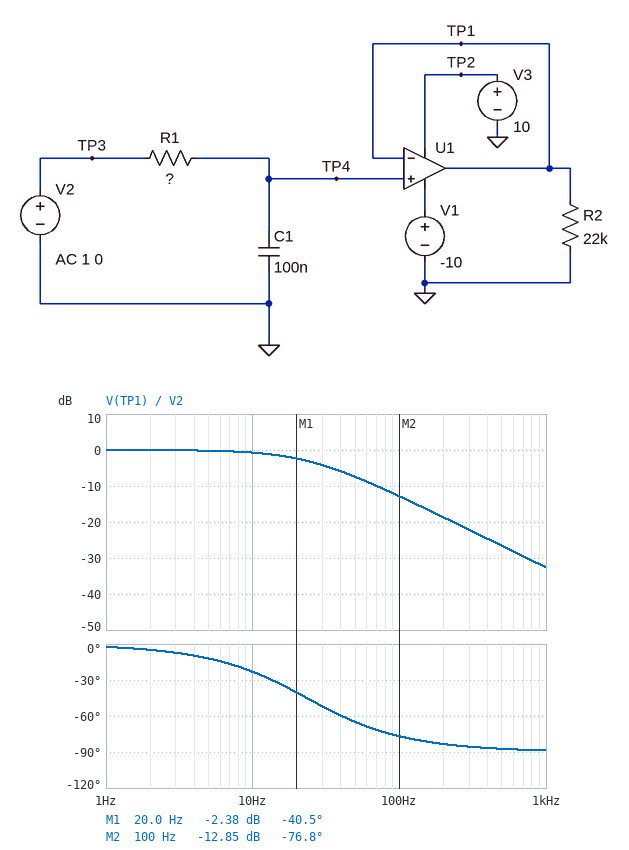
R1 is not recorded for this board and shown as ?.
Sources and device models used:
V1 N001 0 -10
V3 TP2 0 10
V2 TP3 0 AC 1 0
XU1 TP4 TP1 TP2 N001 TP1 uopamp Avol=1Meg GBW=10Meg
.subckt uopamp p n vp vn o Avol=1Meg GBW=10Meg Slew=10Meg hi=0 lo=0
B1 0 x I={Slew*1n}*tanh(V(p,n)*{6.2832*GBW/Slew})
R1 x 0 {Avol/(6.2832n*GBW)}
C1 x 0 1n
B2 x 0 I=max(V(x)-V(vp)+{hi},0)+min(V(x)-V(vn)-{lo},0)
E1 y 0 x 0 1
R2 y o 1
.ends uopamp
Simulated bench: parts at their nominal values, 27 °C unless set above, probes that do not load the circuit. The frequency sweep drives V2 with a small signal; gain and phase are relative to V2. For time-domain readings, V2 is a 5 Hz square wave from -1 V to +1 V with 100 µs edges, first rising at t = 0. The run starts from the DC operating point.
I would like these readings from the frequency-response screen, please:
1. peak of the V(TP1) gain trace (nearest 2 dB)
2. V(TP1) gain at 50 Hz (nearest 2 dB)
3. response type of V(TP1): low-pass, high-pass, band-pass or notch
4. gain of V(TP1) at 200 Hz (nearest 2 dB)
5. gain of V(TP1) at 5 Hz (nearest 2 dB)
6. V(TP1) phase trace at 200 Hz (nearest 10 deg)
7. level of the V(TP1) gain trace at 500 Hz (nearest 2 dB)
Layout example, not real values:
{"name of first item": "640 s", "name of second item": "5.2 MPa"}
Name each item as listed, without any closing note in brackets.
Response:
{"peak of the V(TP1) gain trace": "0 dB", "V(TP1) gain at 50 Hz": "-8 dB", "response type of V(TP1): low-pass, high-pass, band-pass or notch": "low-pass", "gain of V(TP1) at 200 Hz": "-18 dB", "gain of V(TP1) at 5 Hz": "0 dB", "V(TP1) phase trace at 200 Hz": "-80 deg", "level of the V(TP1) gain trace at 500 Hz": "-26 dB"}
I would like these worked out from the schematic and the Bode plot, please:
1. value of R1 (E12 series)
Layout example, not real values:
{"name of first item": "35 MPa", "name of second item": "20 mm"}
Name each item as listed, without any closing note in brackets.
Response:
{"value of R1": "68 kΩ"}
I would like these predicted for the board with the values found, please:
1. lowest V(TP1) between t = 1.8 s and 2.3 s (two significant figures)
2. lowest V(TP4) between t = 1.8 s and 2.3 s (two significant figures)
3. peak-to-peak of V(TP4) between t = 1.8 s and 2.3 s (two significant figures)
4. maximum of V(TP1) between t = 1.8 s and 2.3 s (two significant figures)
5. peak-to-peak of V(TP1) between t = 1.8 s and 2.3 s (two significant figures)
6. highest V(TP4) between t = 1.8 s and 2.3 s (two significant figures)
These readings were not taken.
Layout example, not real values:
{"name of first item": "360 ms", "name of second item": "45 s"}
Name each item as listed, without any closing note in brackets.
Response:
{"lowest V(TP1) between t = 1.8 s and 2.3 s": "-1.0 V", "lowest V(TP4) between t = 1.8 s and 2.3 s": "-1.0 V", "peak-to-peak of V(TP4) between t = 1.8 s and 2.3 s": "2.0 V", "maximum of V(TP1) between t = 1.8 s and 2.3 s": "1.0 V", "peak-to-peak of V(TP1) between t = 1.8 s and 2.3 s": "2.0 V", "highest V(TP4) between t = 1.8 s and 2.3 s": "1.0 V"}
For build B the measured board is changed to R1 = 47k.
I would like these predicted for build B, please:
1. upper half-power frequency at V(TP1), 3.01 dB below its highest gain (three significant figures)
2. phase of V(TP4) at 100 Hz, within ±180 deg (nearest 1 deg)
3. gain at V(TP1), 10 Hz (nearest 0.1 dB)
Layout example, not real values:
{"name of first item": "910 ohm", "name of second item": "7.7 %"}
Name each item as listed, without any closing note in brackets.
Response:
{"upper half-power frequency at V(TP1), 3.01 dB below its highest gain": "33.9 Hz", "phase of V(TP4) at 100 Hz, within ±180 deg": "-71 deg", "gain at V(TP1), 10 Hz": "-0.4 dB"}
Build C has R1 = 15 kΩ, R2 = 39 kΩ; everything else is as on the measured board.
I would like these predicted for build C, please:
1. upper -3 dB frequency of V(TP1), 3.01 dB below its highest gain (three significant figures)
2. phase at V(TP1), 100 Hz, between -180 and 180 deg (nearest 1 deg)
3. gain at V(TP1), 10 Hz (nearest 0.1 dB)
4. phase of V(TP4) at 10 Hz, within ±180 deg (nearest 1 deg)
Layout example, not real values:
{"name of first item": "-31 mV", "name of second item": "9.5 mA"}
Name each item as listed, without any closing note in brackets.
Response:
{"upper -3 dB frequency of V(TP1), 3.01 dB below its highest gain": "106 Hz", "phase at V(TP1), 100 Hz, between -180 and 180 deg": "-43 deg", "gain at V(TP1), 10 Hz": "0 dB", "phase of V(TP4) at 10 Hz, within ±180 deg": "-5 deg"}
